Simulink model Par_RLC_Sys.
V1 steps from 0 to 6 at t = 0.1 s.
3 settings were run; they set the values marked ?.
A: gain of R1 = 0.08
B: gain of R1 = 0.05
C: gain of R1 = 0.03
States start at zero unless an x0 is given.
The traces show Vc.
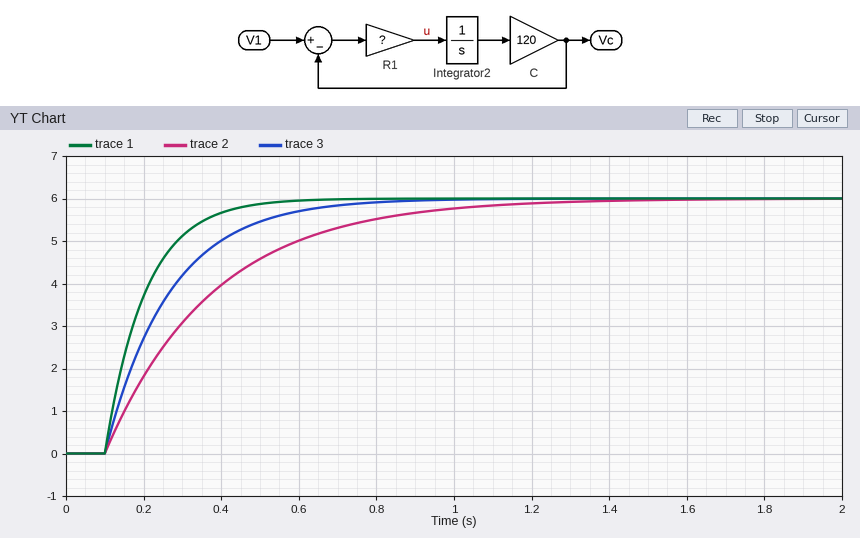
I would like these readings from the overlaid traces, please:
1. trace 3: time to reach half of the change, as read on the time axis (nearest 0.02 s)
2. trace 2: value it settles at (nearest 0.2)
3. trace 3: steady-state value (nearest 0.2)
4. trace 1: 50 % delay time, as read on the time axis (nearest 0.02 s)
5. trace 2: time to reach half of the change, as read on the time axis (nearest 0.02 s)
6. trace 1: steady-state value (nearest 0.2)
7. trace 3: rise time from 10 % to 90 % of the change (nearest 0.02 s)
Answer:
0.22 s
6.0
6.0
0.18 s
0.30 s
6.0
0.36 s
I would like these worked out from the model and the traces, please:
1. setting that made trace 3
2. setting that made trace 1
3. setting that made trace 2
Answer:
B
A
C
